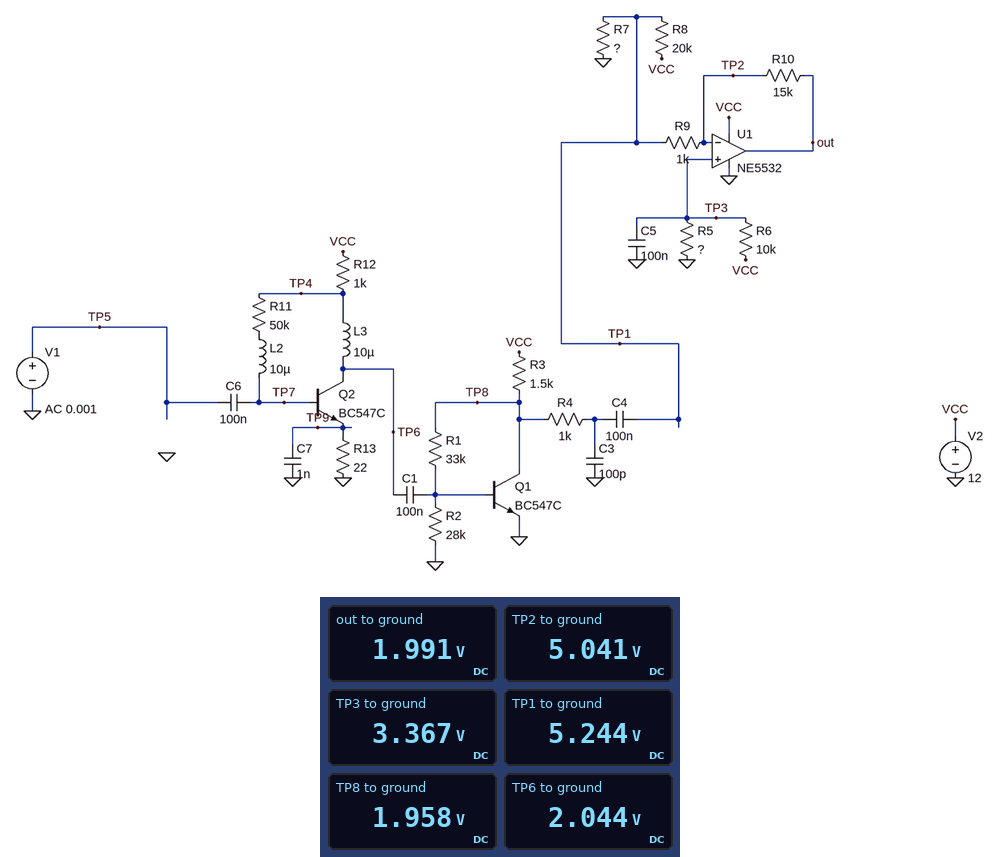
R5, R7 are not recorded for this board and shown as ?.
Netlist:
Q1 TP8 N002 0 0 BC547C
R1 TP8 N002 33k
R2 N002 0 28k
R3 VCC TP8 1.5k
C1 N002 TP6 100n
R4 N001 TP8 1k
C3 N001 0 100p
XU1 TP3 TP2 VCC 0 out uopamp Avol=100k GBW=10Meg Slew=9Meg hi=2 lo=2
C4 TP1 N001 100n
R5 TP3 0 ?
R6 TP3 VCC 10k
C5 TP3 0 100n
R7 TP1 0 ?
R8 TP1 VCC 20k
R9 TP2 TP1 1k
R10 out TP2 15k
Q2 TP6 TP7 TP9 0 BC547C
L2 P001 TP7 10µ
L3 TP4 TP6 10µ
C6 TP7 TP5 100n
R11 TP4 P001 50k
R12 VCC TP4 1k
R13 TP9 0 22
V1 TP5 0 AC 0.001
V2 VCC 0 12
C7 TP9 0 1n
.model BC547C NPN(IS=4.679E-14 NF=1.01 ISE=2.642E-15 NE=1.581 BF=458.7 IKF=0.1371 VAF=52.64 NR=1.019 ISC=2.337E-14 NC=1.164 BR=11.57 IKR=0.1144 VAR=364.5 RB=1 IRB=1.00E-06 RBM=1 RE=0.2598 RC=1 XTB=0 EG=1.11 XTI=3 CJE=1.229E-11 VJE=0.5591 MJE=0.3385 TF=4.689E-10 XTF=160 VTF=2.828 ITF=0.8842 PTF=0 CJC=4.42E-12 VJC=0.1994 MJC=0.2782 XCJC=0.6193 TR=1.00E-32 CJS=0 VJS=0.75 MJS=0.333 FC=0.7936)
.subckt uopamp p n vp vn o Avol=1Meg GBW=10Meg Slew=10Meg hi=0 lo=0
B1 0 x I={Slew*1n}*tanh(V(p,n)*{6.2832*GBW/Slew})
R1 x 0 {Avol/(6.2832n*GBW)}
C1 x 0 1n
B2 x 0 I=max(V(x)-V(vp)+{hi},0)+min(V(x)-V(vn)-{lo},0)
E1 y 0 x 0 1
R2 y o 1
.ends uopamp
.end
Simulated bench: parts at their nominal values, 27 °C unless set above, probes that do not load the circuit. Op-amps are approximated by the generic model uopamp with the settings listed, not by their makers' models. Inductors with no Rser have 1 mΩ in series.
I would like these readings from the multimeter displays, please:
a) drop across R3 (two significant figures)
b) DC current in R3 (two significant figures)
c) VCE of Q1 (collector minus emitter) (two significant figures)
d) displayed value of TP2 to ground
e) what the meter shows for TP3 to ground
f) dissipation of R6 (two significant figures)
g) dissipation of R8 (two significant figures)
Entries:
10 V
6.7 mA
2.0 V
5.041 V
3.367 V
7.5 mW
2.3 mW
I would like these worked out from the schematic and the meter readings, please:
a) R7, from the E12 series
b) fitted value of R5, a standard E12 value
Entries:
39 kΩ
3.9 kΩ
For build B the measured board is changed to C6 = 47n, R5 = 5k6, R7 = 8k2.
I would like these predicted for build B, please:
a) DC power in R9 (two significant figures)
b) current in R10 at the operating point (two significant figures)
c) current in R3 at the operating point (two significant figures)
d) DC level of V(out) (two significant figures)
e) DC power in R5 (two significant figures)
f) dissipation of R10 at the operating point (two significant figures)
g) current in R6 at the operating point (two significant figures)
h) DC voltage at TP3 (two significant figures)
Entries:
14 µW
120 µA
6.7 mA
6.1 V
3.3 mW
220 µW
770 µA
4.3 V
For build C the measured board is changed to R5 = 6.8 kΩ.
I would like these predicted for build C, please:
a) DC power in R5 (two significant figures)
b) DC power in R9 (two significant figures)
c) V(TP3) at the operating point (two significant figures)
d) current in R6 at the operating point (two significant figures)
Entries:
3.5 mW
41 µW
4.9 V
710 µA
